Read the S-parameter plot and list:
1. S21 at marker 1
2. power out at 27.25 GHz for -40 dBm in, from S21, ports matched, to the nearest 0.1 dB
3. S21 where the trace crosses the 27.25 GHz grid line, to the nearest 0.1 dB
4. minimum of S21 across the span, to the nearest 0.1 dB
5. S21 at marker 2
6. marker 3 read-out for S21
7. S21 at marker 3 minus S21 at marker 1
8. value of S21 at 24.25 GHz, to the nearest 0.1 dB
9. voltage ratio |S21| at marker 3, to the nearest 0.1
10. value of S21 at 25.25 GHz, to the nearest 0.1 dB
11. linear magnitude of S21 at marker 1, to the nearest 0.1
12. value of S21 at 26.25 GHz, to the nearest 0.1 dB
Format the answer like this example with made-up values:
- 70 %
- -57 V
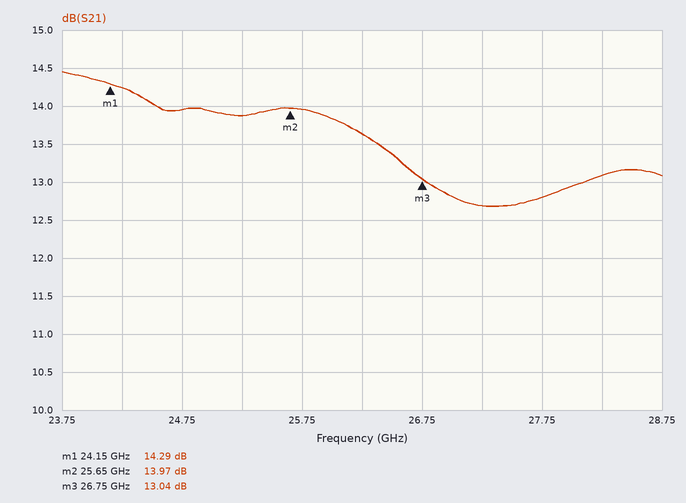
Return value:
- 14.29 dB
- -27.3 dBm
- 12.7 dB
- 12.7 dB
- 13.97 dB
- 13.04 dB
- -1.25 dB
- 14.2 dB
- 4.5
- 13.9 dB
- 5.2
- 13.6 dB
